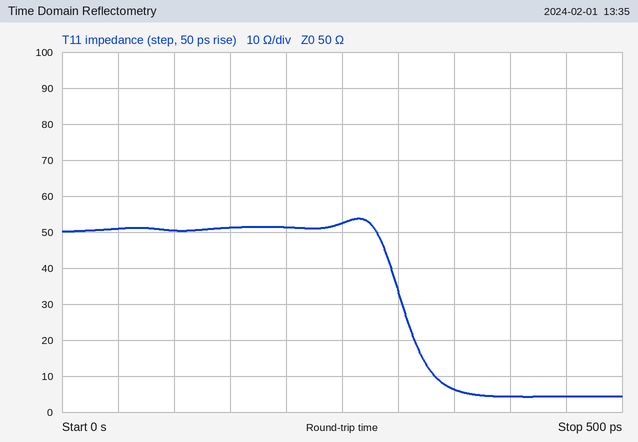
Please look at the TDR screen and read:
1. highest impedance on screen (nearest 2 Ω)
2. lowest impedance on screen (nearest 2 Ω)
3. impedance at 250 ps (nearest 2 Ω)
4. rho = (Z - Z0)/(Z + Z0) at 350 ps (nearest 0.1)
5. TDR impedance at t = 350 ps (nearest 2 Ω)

54 Ω
4 Ω
52 Ω
-0.8
6 Ω
